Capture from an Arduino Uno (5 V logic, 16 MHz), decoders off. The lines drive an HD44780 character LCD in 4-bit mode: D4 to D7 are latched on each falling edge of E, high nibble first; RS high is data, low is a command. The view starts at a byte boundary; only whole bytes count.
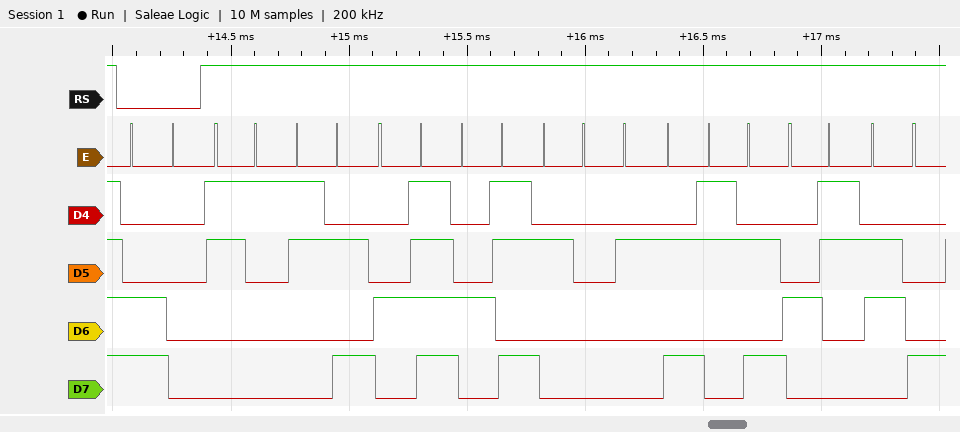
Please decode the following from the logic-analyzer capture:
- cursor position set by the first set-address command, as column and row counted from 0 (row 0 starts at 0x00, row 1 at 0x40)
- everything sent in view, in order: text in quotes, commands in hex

column 0, row 1
0xC0 "1:OK *:Ch"
